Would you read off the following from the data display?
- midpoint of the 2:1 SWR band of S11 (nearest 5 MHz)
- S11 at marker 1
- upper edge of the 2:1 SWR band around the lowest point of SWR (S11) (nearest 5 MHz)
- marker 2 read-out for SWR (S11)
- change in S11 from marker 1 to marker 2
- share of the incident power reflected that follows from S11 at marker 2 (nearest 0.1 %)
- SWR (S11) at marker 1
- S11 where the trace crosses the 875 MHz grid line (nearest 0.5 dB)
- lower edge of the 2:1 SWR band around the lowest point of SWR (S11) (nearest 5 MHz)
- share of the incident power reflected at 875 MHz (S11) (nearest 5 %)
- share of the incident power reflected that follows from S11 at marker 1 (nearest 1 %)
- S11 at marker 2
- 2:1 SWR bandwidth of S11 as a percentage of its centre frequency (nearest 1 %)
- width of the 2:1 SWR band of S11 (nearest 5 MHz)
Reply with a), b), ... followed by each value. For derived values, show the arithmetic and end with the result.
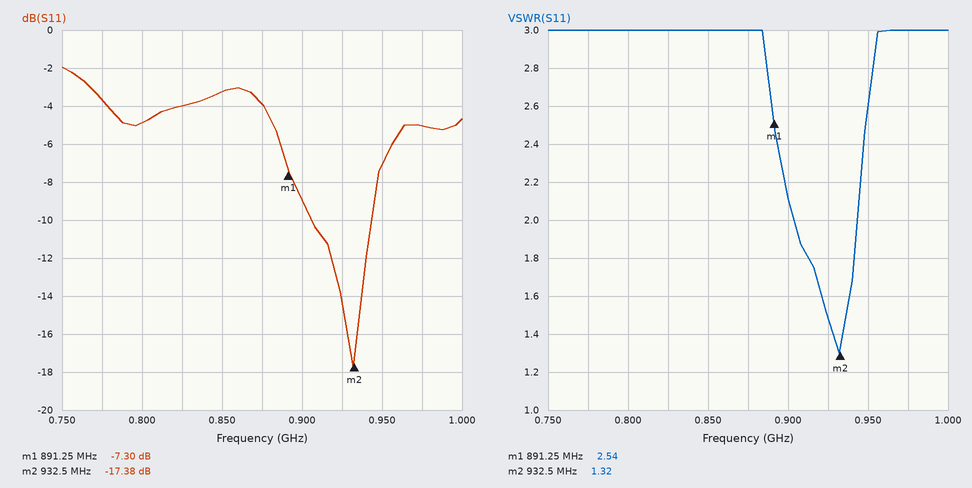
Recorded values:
a) 925 MHz
b) -7.30 dB
c) 945 MHz
d) 1.32
e) -17.38 − (-7.3) = -10.08 dB
f) 10^(-17.38/10) ≈ 1.8 %
g) 2.54
h) -4.0 dB
i) 905 MHz
j) 10^(-4/10) ≈ 40 %
k) 10^(-7.3/10) ≈ 19 %
l) -17.38 dB
m) 40 MHz / 925 MHz ≈ 4 %
n) 945 MHz − 905 MHz = 40 MHz
